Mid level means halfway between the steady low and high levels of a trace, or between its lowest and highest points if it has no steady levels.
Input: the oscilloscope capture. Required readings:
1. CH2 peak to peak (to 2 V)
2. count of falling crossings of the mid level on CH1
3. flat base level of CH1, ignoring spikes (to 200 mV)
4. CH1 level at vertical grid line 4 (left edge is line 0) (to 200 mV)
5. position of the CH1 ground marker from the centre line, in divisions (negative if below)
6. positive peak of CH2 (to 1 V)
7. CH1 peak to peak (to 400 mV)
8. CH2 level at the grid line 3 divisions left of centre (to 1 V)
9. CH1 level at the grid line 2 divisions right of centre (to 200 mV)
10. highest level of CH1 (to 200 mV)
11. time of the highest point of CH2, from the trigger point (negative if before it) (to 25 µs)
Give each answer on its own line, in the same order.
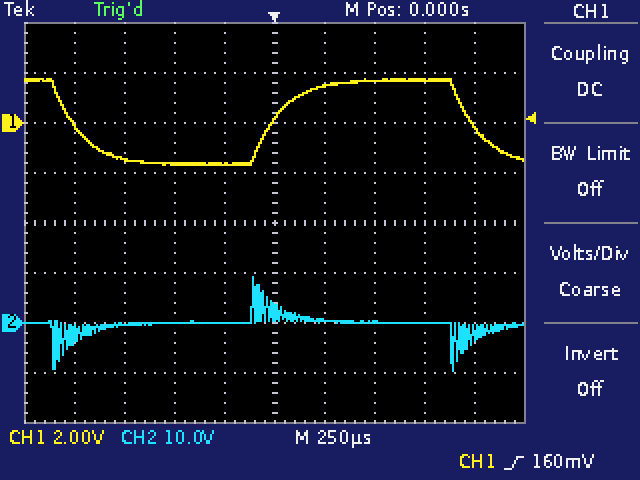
18 V
2
-1.6 V
-1.6 V
+2.0 div
9 V
3.6 V
0 V
1.6 V
1.8 V
-100 µs
